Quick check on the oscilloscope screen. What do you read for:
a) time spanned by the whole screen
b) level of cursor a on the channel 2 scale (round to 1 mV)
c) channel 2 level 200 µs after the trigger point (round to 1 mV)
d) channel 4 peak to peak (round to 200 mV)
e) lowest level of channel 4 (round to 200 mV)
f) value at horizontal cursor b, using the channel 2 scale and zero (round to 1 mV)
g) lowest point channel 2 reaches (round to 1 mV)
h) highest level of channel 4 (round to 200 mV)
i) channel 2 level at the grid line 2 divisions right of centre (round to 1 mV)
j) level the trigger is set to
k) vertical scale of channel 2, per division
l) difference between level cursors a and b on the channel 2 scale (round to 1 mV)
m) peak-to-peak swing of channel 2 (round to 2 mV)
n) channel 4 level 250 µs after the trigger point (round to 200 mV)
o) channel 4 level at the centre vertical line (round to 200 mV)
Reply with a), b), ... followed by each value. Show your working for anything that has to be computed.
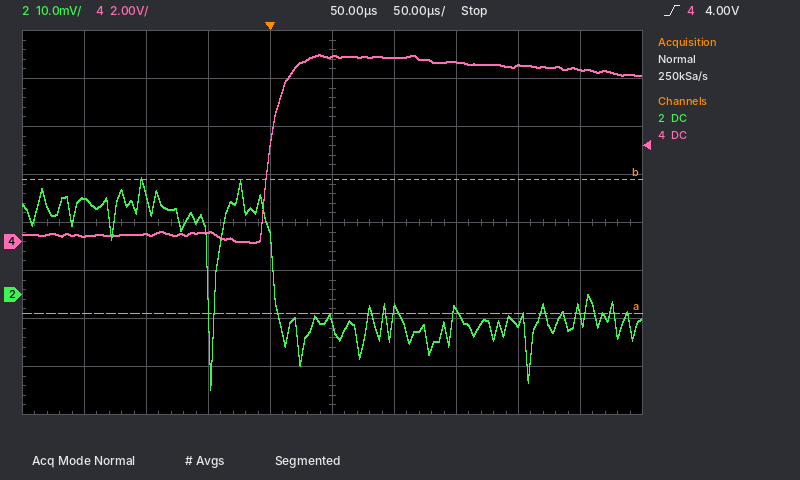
a) 500 µs
b) -4 mV
c) -6 mV
d) 7.8 V − (0.0 V) = 7.8 V
e) 0.0 V
f) 24 mV
g) -20 mV
h) 7.8 V
i) -3 mV
j) 4.00 V
k) 10 mV
l) 28 mV
m) 44 mV
n) 7.2 V
o) 7.8 V
